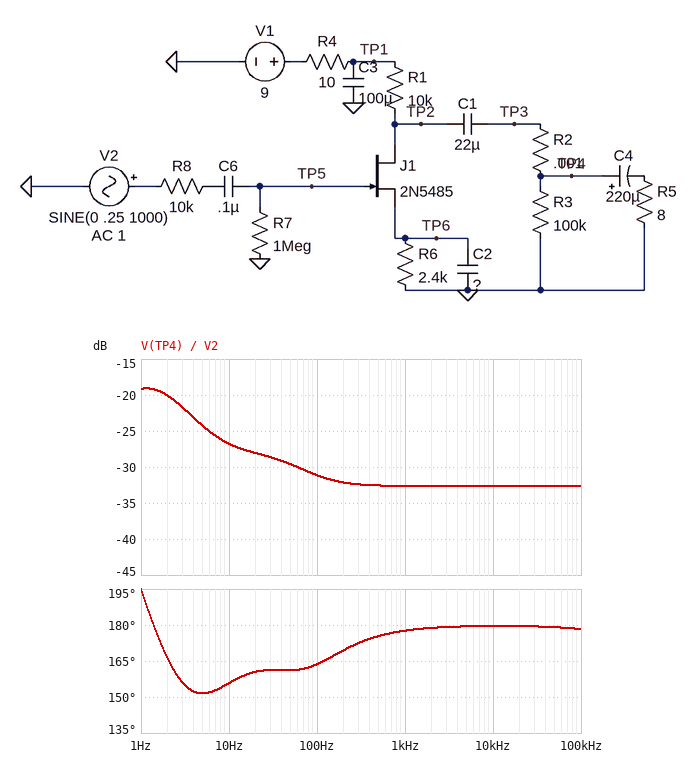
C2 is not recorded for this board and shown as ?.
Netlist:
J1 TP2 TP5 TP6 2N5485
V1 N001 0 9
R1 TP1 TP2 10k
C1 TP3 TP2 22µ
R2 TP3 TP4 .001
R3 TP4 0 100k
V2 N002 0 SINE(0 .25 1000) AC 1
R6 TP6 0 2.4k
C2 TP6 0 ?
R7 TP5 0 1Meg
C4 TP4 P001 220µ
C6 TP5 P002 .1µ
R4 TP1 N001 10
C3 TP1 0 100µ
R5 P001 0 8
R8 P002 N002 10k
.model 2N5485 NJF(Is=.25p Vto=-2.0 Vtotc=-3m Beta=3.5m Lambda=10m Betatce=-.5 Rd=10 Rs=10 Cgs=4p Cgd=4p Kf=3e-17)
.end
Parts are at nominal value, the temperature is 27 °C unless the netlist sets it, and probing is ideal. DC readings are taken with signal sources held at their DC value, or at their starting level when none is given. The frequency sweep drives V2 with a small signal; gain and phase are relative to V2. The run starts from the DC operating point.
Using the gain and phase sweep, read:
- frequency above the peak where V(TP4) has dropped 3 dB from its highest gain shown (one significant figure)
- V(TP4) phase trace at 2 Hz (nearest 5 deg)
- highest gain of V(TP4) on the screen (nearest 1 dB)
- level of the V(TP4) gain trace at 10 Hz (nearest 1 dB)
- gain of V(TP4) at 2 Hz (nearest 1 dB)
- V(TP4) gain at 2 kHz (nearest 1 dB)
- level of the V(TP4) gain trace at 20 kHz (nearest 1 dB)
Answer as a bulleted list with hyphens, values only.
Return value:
- 3 Hz
- 165 deg
- -19 dB
- -27 dB
- -20 dB
- -33 dB
- -33 dB
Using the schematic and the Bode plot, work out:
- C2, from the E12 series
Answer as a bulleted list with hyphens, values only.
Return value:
- 10 µF
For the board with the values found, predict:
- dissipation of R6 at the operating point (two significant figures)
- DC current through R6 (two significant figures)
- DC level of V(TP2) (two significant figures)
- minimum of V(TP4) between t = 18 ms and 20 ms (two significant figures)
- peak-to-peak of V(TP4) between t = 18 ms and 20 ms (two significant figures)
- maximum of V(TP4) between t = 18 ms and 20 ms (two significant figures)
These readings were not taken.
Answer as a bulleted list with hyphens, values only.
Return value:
- 1.0 mW
- 650 µA
- 2.5 V
- -8.5 mV
- 11 mV
- 2.4 mV
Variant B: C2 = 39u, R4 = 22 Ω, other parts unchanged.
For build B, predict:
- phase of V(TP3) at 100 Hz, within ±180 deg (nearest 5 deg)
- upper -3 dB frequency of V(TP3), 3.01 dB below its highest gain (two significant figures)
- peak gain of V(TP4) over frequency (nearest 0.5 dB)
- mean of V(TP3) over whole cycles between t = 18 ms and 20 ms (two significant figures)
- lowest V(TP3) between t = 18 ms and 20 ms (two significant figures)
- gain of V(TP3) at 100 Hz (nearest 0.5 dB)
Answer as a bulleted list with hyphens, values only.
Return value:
- 145 deg
- 15 Hz
- -16.5 dB
- -4.7 mV
- -11 mV
- -30.0 dB
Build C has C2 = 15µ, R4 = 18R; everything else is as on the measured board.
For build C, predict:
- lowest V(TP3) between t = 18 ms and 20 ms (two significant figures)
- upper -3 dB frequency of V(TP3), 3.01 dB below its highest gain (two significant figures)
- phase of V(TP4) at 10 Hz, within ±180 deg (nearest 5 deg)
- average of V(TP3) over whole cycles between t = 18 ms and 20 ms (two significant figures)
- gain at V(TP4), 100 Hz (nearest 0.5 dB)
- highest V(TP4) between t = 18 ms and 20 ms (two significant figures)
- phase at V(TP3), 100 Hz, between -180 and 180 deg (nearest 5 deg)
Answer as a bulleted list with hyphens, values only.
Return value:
- -9.0 mV
- 3.9 Hz
- 160 deg
- -2.8 mV
- -30.5 dB
- 1.9 mV
- 155 deg
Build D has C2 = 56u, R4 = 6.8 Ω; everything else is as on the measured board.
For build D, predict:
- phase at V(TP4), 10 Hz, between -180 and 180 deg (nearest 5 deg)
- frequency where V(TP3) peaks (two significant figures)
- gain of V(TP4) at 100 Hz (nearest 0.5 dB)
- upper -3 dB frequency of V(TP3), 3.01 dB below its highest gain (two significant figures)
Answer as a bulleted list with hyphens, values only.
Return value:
- 145 deg
- 3.5 Hz
- -30.0 dB
- 12 Hz
